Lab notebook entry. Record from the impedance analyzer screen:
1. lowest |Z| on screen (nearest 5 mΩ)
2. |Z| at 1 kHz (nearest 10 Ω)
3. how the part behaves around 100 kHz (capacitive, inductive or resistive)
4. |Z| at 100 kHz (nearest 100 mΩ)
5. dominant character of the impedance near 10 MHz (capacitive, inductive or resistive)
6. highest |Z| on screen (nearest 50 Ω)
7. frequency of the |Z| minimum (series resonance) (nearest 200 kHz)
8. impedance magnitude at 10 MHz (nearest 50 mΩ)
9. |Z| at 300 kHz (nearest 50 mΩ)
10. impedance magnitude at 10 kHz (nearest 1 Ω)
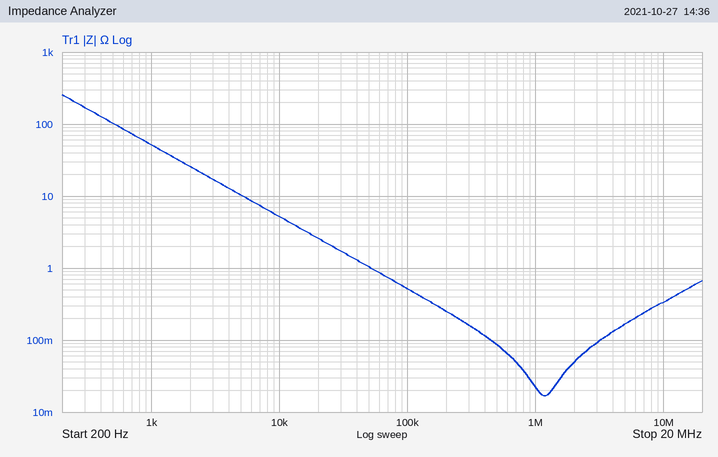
15 mΩ
50 Ω
capacitive
500 mΩ
inductive
250 Ω
1.2 MHz
350 mΩ
150 mΩ
5 Ω
